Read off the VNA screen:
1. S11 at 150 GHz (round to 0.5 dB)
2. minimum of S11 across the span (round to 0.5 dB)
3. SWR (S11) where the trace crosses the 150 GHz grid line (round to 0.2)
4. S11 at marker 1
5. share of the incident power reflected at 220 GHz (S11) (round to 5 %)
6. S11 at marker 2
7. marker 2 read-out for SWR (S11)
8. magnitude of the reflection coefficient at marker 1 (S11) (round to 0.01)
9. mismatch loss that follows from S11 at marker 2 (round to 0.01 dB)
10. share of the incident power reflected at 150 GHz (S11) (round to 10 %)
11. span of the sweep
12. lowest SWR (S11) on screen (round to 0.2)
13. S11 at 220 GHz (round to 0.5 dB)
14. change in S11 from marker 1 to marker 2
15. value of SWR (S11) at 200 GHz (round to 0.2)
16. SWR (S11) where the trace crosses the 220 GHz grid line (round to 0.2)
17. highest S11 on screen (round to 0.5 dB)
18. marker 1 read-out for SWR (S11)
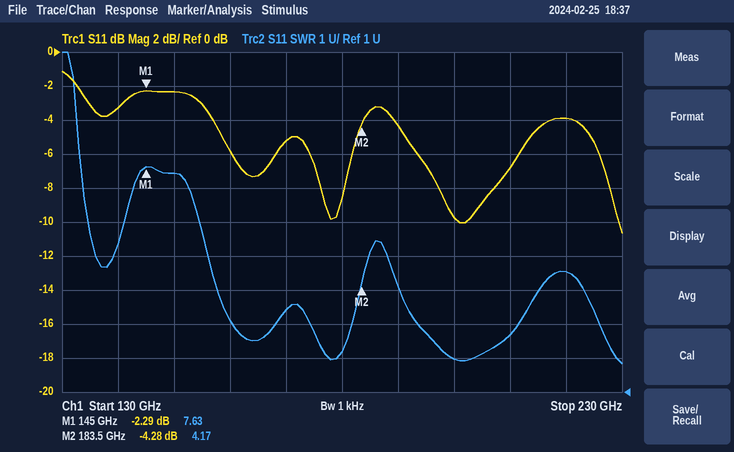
-2.5 dB
-10.5 dB
7.4
-2.29 dB
40 %
-4.28 dB
4.17
0.77
2.03 dB
60 %
100 GHz
1.8
-4.0 dB
-1.99 dB
2.0
4.6
-1.0 dB
7.63
